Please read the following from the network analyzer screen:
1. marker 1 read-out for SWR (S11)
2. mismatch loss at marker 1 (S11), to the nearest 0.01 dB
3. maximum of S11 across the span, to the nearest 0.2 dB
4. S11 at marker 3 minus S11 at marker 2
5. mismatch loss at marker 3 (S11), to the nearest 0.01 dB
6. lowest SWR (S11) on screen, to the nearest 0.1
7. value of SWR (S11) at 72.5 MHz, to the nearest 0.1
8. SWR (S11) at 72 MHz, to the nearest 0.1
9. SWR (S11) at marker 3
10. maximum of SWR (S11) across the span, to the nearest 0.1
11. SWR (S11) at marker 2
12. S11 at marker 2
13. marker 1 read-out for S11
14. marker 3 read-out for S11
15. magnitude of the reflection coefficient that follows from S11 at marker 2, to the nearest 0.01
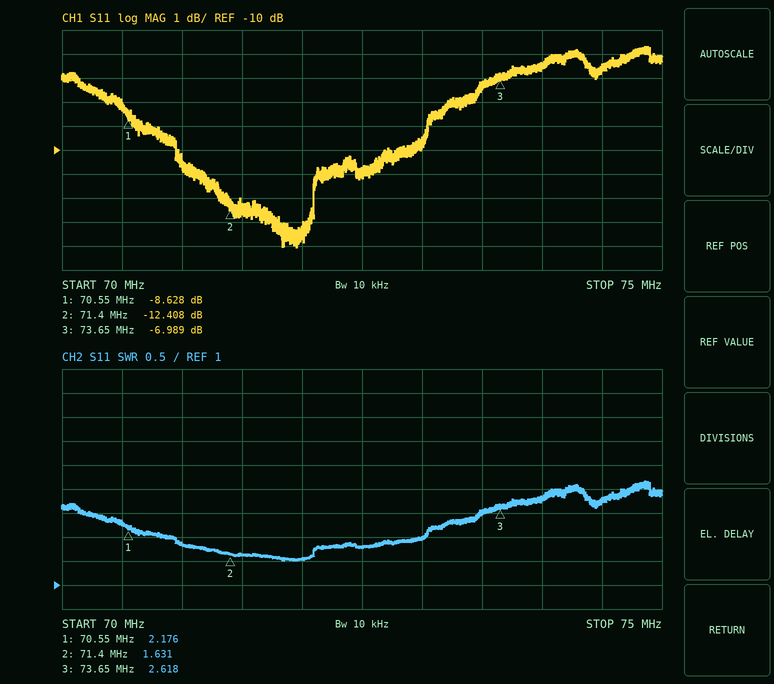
2.176
0.64 dB
-5.6 dB
5.419 dB
0.97 dB
1.5
1.8
1.5
2.618
3.2
1.631
-12.408 dB
-8.628 dB
-6.989 dB
0.24
